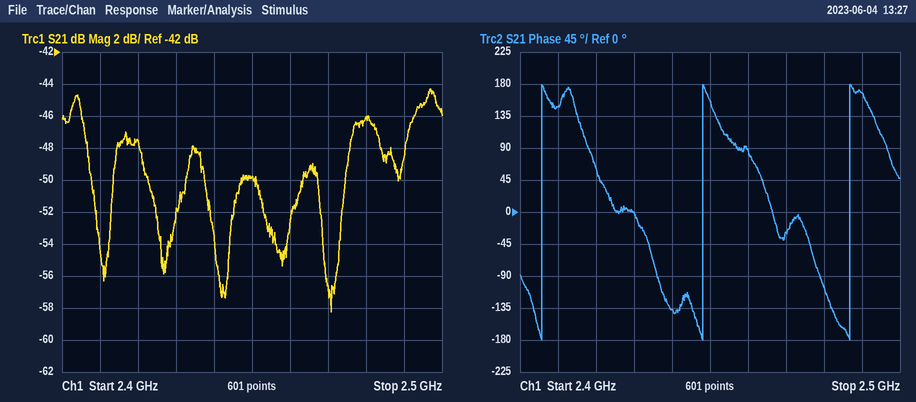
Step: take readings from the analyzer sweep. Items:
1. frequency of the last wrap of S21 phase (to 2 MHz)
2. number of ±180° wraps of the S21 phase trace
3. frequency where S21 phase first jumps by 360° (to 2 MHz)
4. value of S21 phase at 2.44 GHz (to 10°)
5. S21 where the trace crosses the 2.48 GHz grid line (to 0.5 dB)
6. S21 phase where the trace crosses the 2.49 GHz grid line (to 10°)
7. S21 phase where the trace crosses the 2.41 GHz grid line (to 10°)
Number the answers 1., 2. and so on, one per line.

1. 2.486 GHz
2. 3
3. 2.406 GHz
4. -140°
5. -46.0 dB
6. 170°
7. 150°
